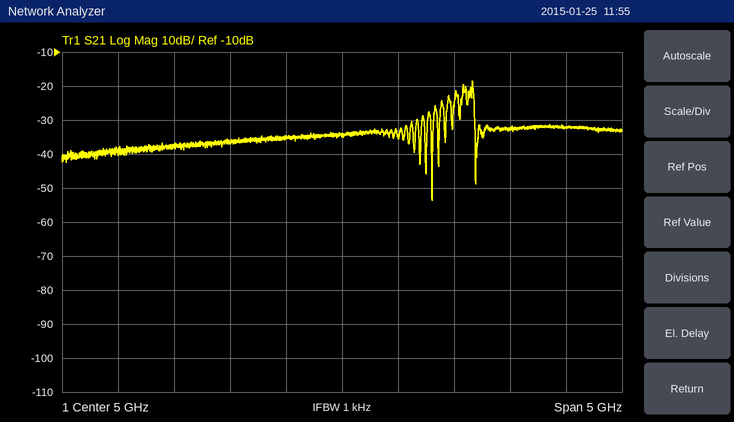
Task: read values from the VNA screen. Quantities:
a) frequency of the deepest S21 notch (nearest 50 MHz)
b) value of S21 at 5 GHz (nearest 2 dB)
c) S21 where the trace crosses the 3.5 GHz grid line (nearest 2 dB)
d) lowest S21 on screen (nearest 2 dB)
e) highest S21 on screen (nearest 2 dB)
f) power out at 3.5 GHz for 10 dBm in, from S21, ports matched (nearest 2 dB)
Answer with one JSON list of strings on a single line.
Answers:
["5.80 GHz", "-34 dB", "-38 dB", "-54 dB", "-18 dB", "-28 dBm"]
